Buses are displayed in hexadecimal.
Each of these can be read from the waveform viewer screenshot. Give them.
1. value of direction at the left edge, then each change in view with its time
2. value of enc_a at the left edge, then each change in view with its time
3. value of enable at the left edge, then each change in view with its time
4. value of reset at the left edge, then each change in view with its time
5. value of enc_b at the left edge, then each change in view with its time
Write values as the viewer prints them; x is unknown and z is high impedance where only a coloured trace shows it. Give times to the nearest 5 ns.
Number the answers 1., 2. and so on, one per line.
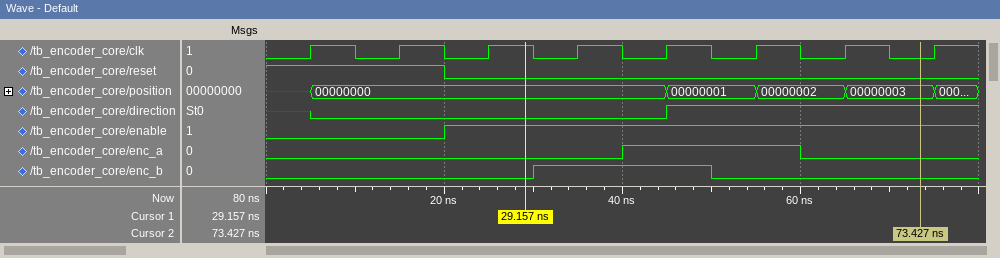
1. x, 0 at 5 ns, 1 at 45 ns
2. 0, 1 at 40 ns, 0 at 60 ns
3. 0, 1 at 20 ns
4. 1, 0 at 20 ns
5. 0, 1 at 30 ns, 0 at 50 ns
